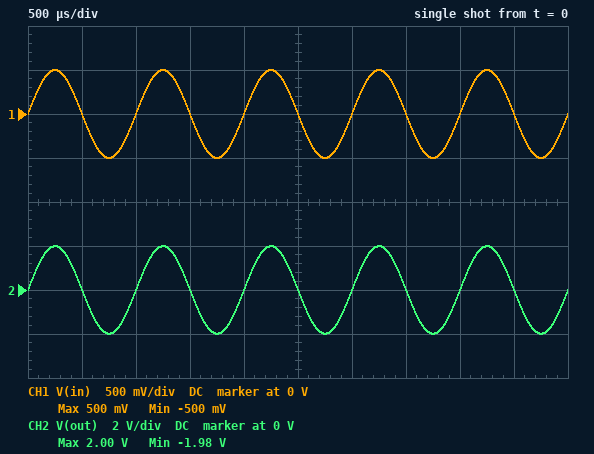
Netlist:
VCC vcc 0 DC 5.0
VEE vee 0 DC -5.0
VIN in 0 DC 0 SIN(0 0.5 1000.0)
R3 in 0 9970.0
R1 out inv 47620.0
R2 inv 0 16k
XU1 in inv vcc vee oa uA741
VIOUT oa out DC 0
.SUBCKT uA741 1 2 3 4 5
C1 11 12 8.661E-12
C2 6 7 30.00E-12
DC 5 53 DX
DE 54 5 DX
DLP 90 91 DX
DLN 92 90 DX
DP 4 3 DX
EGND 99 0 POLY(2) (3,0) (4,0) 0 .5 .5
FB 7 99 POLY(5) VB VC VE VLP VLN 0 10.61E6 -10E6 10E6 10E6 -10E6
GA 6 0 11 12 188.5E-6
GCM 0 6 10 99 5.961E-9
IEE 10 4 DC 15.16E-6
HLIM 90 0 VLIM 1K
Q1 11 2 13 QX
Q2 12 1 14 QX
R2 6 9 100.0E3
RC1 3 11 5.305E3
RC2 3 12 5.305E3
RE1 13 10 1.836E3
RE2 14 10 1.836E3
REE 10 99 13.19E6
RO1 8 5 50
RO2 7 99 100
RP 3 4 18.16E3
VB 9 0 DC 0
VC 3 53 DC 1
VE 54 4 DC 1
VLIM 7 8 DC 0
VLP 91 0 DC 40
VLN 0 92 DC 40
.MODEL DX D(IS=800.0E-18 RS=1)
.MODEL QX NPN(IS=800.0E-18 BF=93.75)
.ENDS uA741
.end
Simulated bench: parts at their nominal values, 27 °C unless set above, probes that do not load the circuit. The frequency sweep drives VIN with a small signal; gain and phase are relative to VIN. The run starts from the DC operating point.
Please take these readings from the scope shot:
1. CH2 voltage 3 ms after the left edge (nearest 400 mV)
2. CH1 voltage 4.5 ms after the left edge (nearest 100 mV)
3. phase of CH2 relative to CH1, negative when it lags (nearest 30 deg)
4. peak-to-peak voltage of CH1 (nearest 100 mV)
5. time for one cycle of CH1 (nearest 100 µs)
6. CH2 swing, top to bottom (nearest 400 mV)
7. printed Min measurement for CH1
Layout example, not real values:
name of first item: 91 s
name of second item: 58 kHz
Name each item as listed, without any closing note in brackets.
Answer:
CH2 voltage 3 ms after the left edge: 0 V
CH1 voltage 4.5 ms after the left edge: 0 V
phase of CH2 relative to CH1, negative when it lags: 0 deg
peak-to-peak voltage of CH1: 1.0 V
time for one cycle of CH1: 1.0 ms
CH2 swing, top to bottom: 4.0 V
printed Min measurement for CH1: -500 mV
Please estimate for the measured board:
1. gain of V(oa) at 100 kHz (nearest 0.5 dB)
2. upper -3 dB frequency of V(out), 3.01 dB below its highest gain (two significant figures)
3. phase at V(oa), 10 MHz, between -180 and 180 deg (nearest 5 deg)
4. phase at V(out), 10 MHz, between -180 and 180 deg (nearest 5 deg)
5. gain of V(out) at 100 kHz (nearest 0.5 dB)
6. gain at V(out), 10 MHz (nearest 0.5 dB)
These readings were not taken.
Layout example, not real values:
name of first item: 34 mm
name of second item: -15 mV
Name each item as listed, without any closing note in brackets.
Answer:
gain of V(oa) at 100 kHz: 11.5 dB
upper -3 dB frequency of V(out), 3.01 dB below its highest gain: 290 kHz
phase at V(oa), 10 MHz, between -180 and 180 deg: -170 deg
phase at V(out), 10 MHz, between -180 and 180 deg: -170 deg
gain of V(out) at 100 kHz: 11.5 dB
gain at V(out), 10 MHz: -35.5 dB
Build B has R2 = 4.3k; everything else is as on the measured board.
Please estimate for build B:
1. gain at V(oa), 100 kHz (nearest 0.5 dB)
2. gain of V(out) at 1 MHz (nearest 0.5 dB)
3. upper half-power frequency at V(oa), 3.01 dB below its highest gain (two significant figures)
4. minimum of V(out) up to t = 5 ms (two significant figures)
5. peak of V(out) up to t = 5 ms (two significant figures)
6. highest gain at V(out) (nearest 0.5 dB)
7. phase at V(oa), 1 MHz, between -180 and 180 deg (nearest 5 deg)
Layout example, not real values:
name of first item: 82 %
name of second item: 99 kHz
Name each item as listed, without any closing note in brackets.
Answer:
gain at V(oa), 100 kHz: 18.0 dB
gain of V(out) at 1 MHz: -1.0 dB
upper half-power frequency at V(oa), 3.01 dB below its highest gain: 86 kHz
minimum of V(out) up to t = 5 ms: -4.6 V
peak of V(out) up to t = 5 ms: 4.6 V
highest gain at V(out): 21.5 dB
phase at V(oa), 1 MHz, between -180 and 180 deg: -115 deg
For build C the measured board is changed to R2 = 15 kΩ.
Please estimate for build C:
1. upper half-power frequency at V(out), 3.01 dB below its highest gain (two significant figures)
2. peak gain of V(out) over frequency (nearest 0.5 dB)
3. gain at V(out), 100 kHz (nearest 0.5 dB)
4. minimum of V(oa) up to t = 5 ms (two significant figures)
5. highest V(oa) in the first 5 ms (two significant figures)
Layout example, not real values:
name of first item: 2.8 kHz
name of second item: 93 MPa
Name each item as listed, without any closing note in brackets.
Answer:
upper half-power frequency at V(out), 3.01 dB below its highest gain: 270 kHz
peak gain of V(out) over frequency: 12.5 dB
gain at V(out), 100 kHz: 12.0 dB
minimum of V(oa) up to t = 5 ms: -2.1 V
highest V(oa) in the first 5 ms: 2.1 V
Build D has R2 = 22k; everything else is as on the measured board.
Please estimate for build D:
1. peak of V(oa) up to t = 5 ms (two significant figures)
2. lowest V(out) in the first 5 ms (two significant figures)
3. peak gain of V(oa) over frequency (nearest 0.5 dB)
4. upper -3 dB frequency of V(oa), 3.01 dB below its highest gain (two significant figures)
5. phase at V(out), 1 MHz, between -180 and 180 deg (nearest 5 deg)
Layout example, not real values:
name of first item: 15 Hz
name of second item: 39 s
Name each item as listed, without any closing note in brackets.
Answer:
peak of V(oa) up to t = 5 ms: 1.6 V
lowest V(out) in the first 5 ms: -1.6 V
peak gain of V(oa) over frequency: 10.0 dB
upper -3 dB frequency of V(oa), 3.01 dB below its highest gain: 370 kHz
phase at V(out), 1 MHz, between -180 and 180 deg: -105 deg
